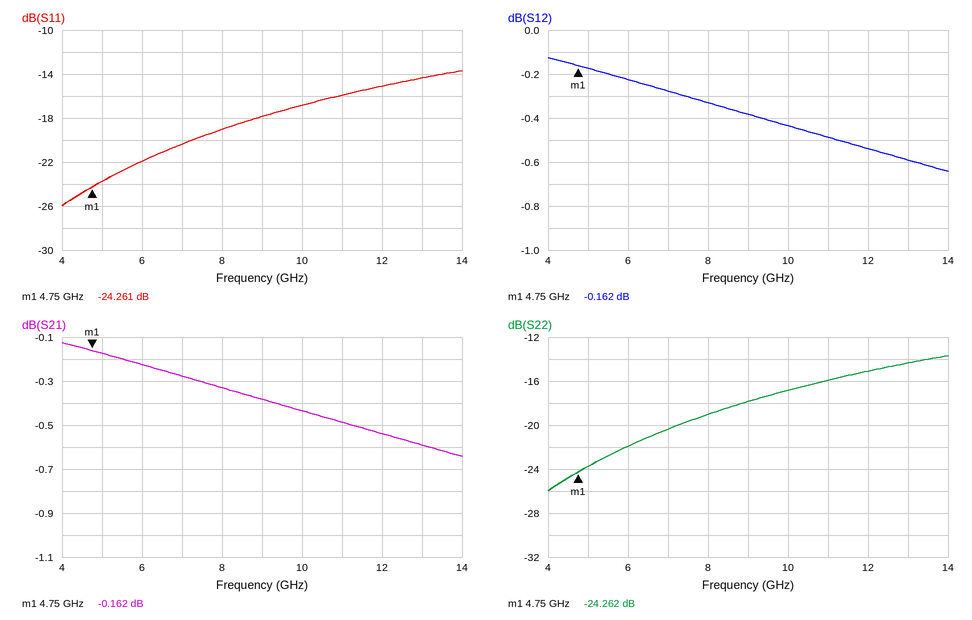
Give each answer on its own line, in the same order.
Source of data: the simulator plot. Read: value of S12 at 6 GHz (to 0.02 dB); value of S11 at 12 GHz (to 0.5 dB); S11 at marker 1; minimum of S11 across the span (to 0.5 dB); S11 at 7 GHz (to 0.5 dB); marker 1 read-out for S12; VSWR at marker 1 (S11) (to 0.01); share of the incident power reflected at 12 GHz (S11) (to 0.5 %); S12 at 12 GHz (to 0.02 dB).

-0.22 dB
-15.0 dB
-24.261 dB
-26.0 dB
-20.5 dB
-0.162 dB
1.13
3.0 %
-0.54 dB
